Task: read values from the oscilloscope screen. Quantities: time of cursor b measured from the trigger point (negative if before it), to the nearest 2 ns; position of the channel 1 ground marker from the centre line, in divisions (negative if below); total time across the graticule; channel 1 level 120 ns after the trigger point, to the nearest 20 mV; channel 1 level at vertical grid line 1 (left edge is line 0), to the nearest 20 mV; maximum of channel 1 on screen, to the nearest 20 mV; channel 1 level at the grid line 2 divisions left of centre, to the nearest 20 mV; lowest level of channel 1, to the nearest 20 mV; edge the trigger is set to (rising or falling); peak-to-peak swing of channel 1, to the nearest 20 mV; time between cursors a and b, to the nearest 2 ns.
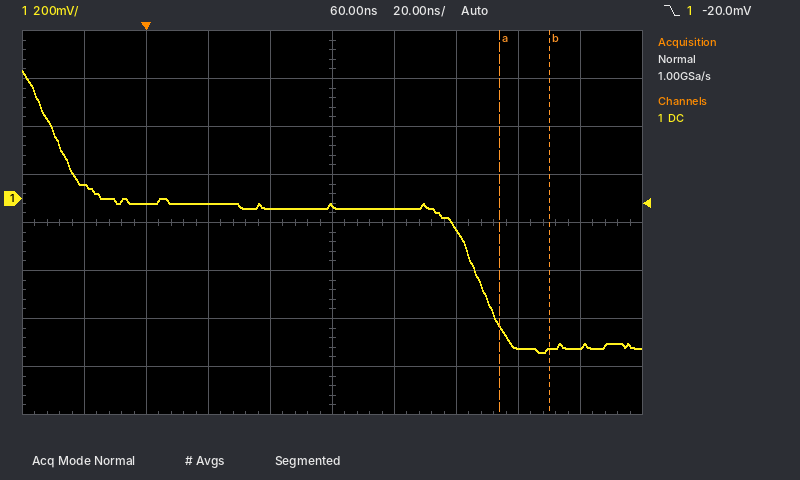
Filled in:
+130 ns
+0.5 div
200 ns
-620 mV
60 mV
540 mV
-20 mV
-640 mV
falling
1.18 V
16 ns
